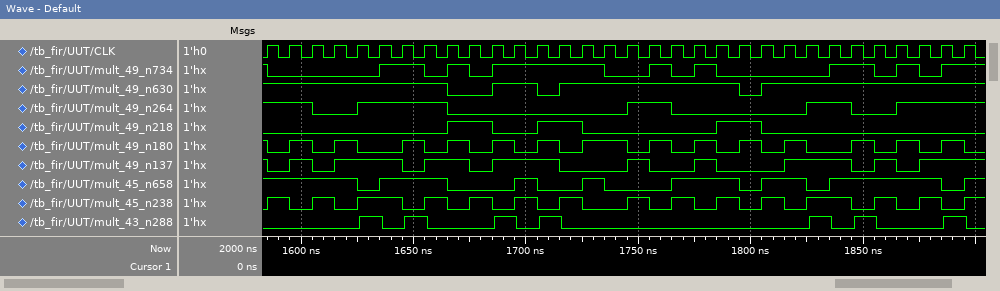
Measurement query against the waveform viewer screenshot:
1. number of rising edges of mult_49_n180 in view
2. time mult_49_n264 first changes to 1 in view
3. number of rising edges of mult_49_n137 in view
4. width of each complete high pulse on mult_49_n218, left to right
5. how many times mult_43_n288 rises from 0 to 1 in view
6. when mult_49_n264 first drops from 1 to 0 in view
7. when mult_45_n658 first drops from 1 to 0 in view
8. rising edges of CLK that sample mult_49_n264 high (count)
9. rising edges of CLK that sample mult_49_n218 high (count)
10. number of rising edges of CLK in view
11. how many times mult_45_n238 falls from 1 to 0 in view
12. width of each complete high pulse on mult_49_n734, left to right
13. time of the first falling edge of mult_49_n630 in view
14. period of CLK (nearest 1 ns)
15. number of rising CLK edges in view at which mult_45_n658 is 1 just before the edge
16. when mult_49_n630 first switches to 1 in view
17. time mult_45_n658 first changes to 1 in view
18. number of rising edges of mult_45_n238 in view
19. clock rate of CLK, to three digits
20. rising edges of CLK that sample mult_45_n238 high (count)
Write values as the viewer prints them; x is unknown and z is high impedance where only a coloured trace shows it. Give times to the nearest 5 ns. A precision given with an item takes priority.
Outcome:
14
1625 ns
9
20 ns, 20 ns, 20 ns
7
1605 ns
1625 ns
14
6
32
14
20 ns, 10 ns, 50 ns, 10 ns, 10 ns, 20 ns, 10 ns
1665 ns
10 ns
20
1685 ns
1635 ns
15
100 MHz
16
